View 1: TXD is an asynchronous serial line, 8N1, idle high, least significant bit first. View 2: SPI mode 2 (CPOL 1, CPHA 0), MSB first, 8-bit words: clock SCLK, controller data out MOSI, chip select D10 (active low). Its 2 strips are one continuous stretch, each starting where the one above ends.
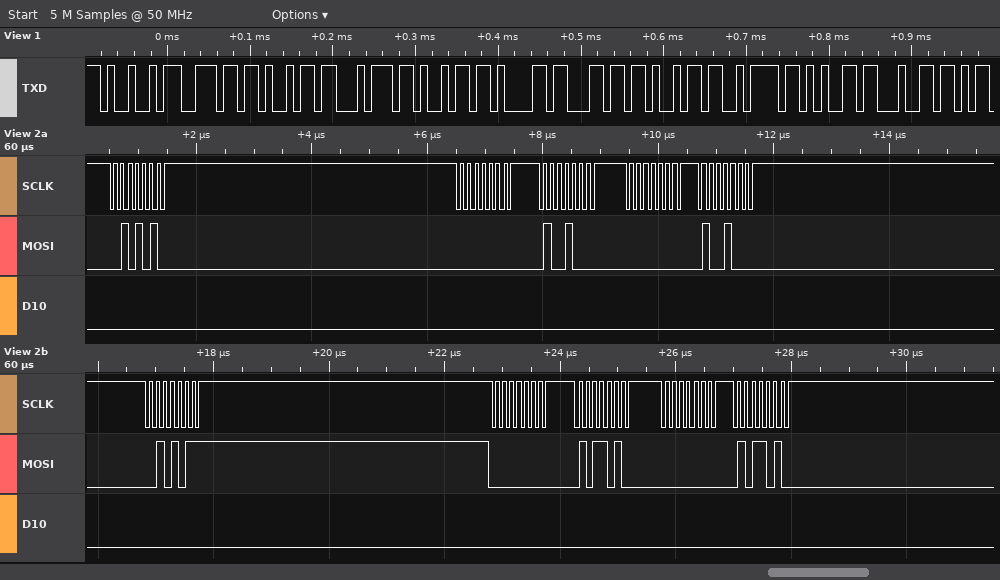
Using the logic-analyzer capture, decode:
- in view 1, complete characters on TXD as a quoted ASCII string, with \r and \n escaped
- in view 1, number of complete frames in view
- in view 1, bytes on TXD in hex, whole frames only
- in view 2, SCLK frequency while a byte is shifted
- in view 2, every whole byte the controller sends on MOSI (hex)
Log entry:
"Initialized"
11
49 6E 69 74 69 61 6C 69 7A 65 64
8 MHz
2A 00 48 00 48 2B 00 5A 00 5A
